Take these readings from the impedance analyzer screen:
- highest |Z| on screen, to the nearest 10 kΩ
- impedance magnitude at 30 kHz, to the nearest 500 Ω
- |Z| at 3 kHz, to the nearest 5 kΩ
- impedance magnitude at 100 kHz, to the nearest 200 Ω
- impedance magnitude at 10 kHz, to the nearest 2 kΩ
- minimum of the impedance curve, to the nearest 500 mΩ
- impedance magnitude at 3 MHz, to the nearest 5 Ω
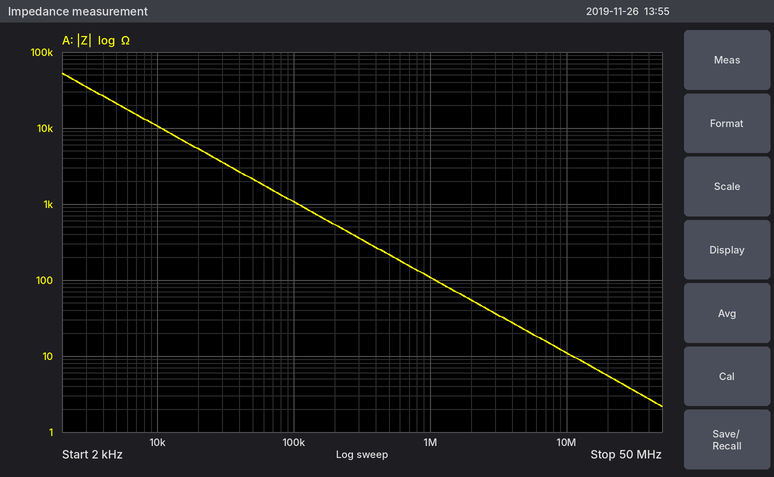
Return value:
50 kΩ
3.5 kΩ
35 kΩ
1.0 kΩ
10 kΩ
2.0 Ω
35 Ω
